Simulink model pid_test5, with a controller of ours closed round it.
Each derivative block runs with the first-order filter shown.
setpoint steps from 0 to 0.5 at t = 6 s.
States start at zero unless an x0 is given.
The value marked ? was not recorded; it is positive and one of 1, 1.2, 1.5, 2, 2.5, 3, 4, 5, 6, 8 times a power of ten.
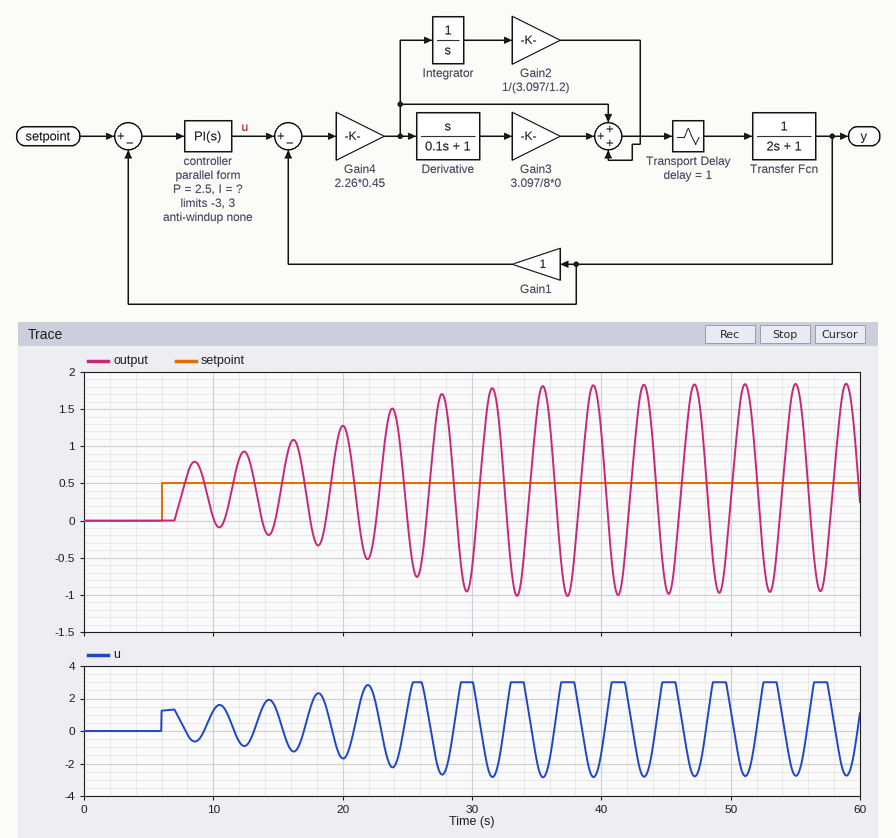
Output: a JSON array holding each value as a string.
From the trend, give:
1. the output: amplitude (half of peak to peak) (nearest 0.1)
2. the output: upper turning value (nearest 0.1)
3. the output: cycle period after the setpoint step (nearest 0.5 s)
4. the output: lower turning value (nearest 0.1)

["1.4", "1.8", "4.0 s", "-1.0"]
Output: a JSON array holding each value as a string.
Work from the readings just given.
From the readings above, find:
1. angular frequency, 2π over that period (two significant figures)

["1.6 rad/s"]
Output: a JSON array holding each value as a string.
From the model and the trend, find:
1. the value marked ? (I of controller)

["0.15"]
